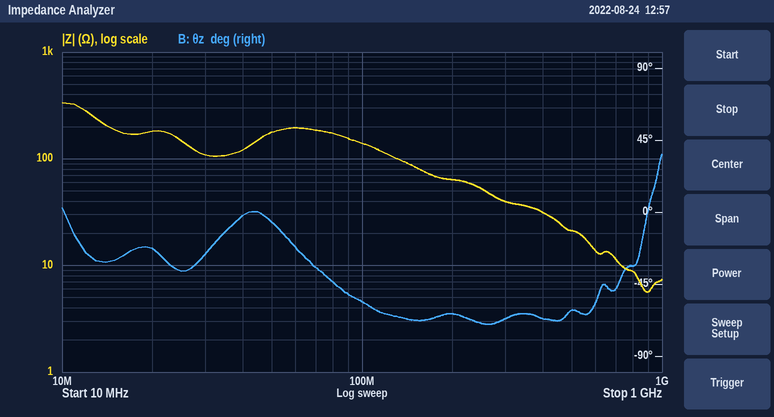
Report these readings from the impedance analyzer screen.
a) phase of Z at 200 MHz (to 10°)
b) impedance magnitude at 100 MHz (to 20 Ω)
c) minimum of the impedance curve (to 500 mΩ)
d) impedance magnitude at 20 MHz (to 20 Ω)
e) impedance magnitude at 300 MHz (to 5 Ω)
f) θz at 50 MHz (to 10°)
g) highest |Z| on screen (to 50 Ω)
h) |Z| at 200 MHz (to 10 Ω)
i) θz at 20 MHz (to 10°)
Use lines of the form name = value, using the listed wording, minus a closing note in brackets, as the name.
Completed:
phase of Z at 200 MHz = -60°
impedance magnitude at 100 MHz = 140 Ω
minimum of the impedance curve = 5.5 Ω
impedance magnitude at 20 MHz = 180 Ω
impedance magnitude at 300 MHz = 40 Ω
θz at 50 MHz = -10°
highest |Z| on screen = 350 Ω
|Z| at 200 MHz = 60 Ω
θz at 20 MHz = -20°
